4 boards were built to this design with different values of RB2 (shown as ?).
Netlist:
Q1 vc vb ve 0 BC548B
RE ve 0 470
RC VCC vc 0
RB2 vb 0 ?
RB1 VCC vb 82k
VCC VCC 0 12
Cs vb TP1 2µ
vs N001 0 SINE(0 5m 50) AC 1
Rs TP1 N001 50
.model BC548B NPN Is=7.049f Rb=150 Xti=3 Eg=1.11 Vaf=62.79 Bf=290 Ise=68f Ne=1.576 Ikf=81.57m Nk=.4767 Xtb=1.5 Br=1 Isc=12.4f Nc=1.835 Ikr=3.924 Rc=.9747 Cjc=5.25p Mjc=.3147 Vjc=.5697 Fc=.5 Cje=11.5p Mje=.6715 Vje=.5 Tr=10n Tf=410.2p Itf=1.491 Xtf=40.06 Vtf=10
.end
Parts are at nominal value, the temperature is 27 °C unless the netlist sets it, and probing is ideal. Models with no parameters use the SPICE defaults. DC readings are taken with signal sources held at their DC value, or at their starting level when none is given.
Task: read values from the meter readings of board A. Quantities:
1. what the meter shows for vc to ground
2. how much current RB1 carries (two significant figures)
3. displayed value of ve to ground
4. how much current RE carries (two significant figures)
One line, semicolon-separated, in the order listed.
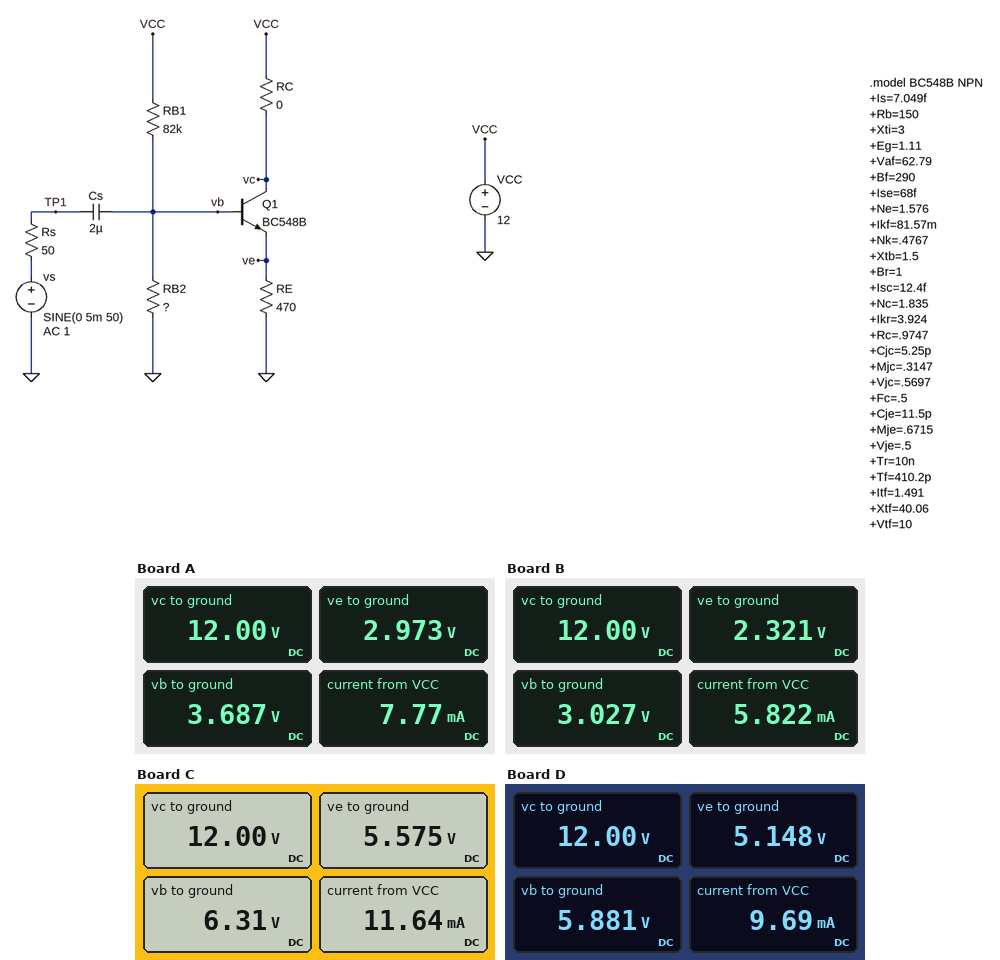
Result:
12.00 V; 100 µA; 2.973 V; 6.3 mA
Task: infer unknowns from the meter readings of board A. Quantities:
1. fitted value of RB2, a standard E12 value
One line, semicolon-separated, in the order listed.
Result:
47 kΩ
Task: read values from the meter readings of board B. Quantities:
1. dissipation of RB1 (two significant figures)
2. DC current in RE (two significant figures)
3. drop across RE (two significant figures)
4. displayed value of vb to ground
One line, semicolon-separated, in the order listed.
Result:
980 µW; 4.9 mA; 2.3 V; 3.027 V
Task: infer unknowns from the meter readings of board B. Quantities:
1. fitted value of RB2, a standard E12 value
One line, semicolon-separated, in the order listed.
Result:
33 kΩ
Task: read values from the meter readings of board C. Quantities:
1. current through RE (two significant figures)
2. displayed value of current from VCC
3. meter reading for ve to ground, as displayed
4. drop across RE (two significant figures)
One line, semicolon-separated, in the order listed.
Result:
12 mA; 11.64 mA; 5.575 V; 5.6 V
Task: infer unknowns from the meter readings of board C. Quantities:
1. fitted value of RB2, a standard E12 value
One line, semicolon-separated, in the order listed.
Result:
270 kΩ
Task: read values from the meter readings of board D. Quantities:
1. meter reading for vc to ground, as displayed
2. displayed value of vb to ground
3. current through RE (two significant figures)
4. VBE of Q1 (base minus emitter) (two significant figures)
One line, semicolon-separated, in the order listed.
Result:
12.00 V; 5.881 V; 11 mA; 730 mV
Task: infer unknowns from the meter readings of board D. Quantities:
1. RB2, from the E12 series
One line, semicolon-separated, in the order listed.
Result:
180 kΩ
